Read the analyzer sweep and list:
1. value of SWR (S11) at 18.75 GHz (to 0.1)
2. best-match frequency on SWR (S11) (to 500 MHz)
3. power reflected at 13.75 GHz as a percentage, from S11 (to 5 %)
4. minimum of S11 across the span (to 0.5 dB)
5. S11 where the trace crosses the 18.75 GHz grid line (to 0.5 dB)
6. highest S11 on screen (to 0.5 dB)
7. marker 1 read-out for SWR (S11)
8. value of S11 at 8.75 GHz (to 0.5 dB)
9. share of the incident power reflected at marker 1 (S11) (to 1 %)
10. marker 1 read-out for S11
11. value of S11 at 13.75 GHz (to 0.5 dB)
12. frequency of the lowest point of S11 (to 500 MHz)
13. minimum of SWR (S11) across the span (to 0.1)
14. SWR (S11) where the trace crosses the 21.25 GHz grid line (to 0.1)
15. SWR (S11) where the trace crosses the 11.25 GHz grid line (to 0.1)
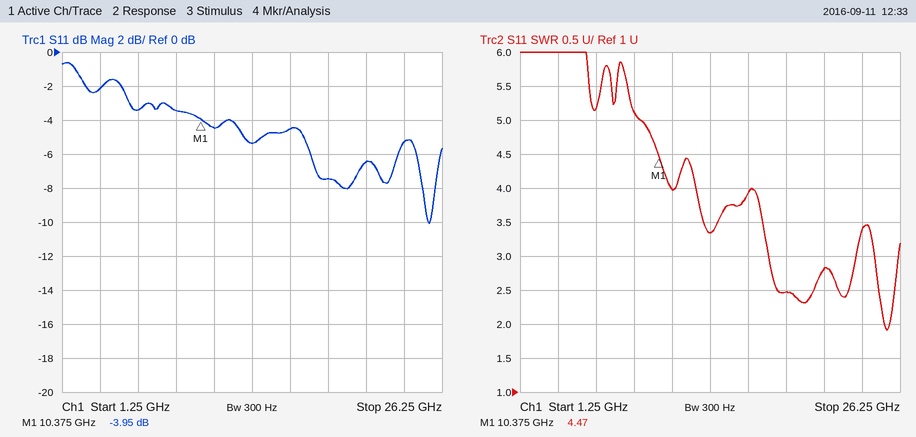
2.5
25.5 GHz
30 %
-10.0 dB
-7.5 dB
-0.5 dB
4.47
-3.5 dB
40 %
-3.95 dB
-5.5 dB
25.5 GHz
1.9
2.8
4.0
